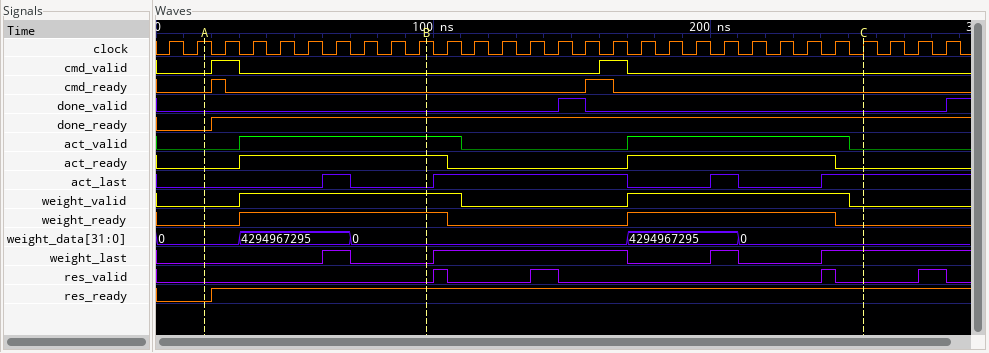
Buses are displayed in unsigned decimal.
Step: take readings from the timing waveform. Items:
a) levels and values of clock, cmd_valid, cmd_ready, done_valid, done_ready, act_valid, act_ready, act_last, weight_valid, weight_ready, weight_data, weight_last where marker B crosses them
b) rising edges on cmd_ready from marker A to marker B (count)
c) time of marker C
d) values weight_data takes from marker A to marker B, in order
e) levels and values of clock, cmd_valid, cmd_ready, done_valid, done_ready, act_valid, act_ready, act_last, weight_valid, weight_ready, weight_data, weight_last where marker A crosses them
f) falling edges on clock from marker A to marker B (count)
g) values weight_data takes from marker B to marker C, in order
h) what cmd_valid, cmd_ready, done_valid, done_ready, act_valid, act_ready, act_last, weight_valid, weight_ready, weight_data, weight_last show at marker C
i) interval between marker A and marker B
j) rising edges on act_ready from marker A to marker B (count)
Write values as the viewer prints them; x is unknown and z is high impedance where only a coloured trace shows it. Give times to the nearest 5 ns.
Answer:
clock=1, cmd_valid=0, cmd_ready=0, done_valid=0, done_ready=1, act_valid=1, act_ready=1, act_last=0, weight_valid=1, weight_ready=1, weight_data=0, weight_last=0
1
255 ns
0, 4294967295, 0
clock=1, cmd_valid=0, cmd_ready=0, done_valid=0, done_ready=0, act_valid=0, act_ready=0, act_last=0, weight_valid=0, weight_ready=0, weight_data=0, weight_last=0
8
0, 4294967295, 0
cmd_valid=0, cmd_ready=0, done_valid=0, done_ready=1, act_valid=0, act_ready=0, act_last=1, weight_valid=0, weight_ready=0, weight_data=0, weight_last=1
80 ns
1
